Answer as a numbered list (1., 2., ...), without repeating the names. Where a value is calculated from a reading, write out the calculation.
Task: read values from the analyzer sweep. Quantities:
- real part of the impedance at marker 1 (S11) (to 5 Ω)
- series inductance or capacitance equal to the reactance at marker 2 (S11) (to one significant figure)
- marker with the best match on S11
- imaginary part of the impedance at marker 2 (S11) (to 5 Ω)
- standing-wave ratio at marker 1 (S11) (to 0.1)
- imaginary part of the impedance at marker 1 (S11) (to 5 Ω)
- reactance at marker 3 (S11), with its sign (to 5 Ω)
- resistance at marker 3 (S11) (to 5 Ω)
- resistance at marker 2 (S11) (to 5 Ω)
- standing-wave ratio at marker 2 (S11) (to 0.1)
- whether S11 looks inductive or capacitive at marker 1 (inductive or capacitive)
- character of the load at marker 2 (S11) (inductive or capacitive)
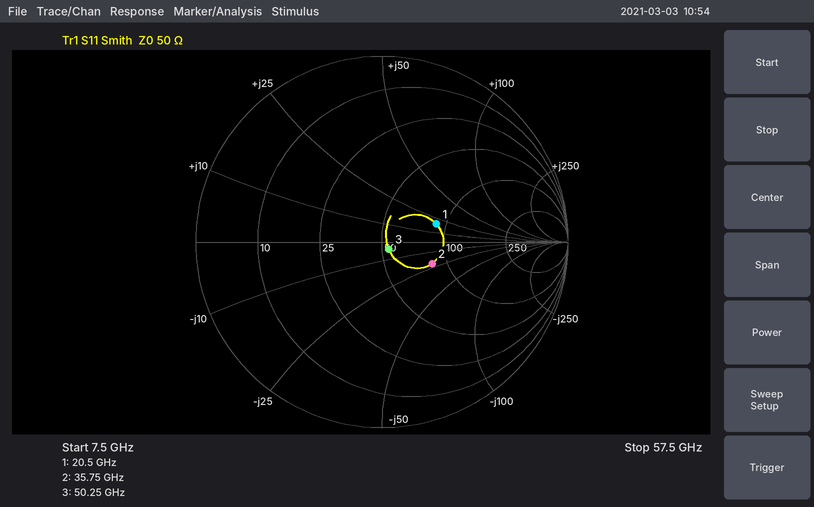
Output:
1. 90 Ω
2. C = 1/(2π × 35.75 GHz × 20 Ω) ≈ 223 fF, so 200 fF to one significant figure
3. marker 3
4. -20 Ω
5. 1.9
6. +20 Ω
7. -5 Ω
8. 55 Ω
9. 85 Ω
10. 1.8
11. inductive
12. capacitive
